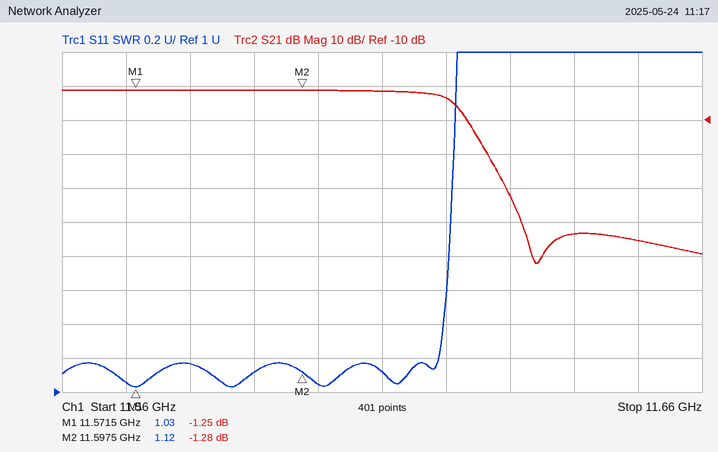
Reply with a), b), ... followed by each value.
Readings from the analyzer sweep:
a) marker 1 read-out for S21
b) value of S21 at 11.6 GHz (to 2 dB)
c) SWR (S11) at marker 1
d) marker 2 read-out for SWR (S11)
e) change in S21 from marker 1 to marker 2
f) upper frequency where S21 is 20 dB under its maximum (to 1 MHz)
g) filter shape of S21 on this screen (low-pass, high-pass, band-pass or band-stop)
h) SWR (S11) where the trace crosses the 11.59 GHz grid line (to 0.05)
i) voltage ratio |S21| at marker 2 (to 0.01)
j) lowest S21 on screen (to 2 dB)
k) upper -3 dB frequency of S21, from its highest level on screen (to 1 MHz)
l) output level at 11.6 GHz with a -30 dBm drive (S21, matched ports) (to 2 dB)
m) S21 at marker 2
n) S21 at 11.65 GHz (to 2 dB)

a) -1.25 dB
b) -2 dB
c) 1.03
d) 1.12
e) -0.03 dB
f) 11.627 GHz
g) low-pass
h) 1.10
i) 0.86
j) -52 dB
k) 11.621 GHz
l) -32 dBm
m) -1.28 dB
n) -46 dB
